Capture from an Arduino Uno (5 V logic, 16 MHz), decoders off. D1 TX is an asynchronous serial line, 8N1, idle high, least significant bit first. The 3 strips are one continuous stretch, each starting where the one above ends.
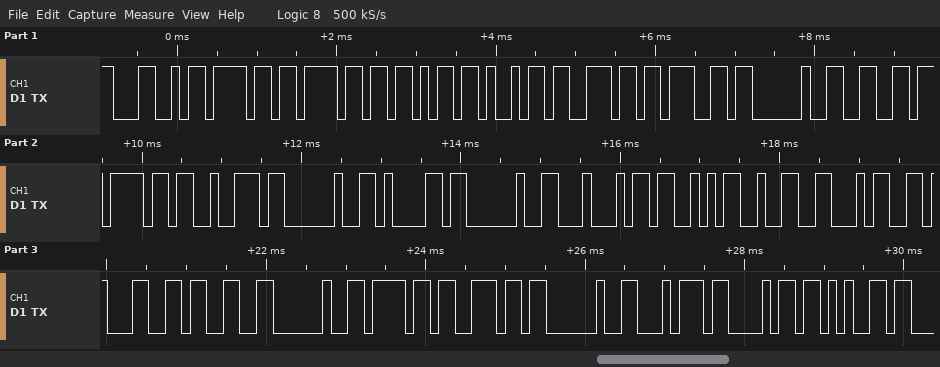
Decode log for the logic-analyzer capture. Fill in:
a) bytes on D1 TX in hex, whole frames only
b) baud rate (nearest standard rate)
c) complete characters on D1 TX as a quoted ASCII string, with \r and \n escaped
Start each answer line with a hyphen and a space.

- 4C 6F 6F 6B 69 6E 67 20 66 6F 72 20 61 20 44 53 32 34 31 33 20 6F 6E 20 74 68 65
- 9600 baud
- "Looking for a DS2413 on the"
